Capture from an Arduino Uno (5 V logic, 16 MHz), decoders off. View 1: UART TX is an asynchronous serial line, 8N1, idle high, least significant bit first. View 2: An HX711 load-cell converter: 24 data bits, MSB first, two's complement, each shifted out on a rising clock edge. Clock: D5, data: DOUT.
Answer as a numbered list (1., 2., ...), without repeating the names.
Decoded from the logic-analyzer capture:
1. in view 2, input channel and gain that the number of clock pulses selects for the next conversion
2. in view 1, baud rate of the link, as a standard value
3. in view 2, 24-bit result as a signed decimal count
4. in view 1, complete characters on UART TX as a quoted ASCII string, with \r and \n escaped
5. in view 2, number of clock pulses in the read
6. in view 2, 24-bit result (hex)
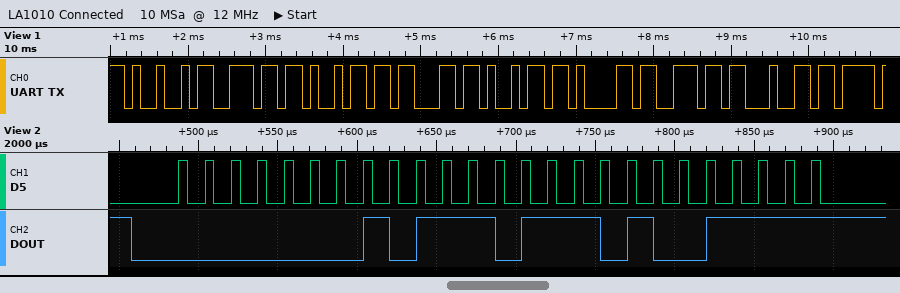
1. channel A, gain 128
2. 9600 baud
3. 96079
4. "Iniciand"
5. 25
6. 0x01774F
